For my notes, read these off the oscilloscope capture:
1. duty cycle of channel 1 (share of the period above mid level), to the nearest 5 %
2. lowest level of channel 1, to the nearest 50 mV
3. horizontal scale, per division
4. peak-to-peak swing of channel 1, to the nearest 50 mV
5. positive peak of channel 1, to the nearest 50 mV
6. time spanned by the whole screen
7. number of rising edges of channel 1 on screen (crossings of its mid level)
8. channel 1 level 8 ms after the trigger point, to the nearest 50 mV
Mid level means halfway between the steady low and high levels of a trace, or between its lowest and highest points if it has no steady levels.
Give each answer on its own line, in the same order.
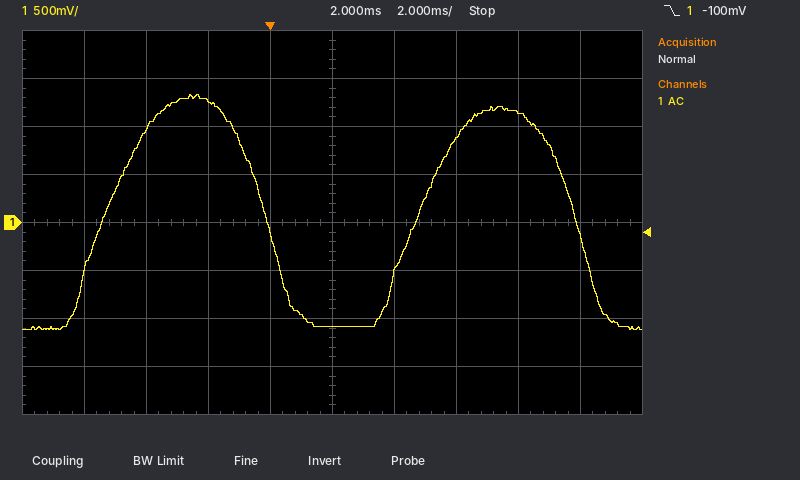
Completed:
50 %
-1.10 V
2 ms
2.45 V
1.35 V
20 ms
2
1.15 V
